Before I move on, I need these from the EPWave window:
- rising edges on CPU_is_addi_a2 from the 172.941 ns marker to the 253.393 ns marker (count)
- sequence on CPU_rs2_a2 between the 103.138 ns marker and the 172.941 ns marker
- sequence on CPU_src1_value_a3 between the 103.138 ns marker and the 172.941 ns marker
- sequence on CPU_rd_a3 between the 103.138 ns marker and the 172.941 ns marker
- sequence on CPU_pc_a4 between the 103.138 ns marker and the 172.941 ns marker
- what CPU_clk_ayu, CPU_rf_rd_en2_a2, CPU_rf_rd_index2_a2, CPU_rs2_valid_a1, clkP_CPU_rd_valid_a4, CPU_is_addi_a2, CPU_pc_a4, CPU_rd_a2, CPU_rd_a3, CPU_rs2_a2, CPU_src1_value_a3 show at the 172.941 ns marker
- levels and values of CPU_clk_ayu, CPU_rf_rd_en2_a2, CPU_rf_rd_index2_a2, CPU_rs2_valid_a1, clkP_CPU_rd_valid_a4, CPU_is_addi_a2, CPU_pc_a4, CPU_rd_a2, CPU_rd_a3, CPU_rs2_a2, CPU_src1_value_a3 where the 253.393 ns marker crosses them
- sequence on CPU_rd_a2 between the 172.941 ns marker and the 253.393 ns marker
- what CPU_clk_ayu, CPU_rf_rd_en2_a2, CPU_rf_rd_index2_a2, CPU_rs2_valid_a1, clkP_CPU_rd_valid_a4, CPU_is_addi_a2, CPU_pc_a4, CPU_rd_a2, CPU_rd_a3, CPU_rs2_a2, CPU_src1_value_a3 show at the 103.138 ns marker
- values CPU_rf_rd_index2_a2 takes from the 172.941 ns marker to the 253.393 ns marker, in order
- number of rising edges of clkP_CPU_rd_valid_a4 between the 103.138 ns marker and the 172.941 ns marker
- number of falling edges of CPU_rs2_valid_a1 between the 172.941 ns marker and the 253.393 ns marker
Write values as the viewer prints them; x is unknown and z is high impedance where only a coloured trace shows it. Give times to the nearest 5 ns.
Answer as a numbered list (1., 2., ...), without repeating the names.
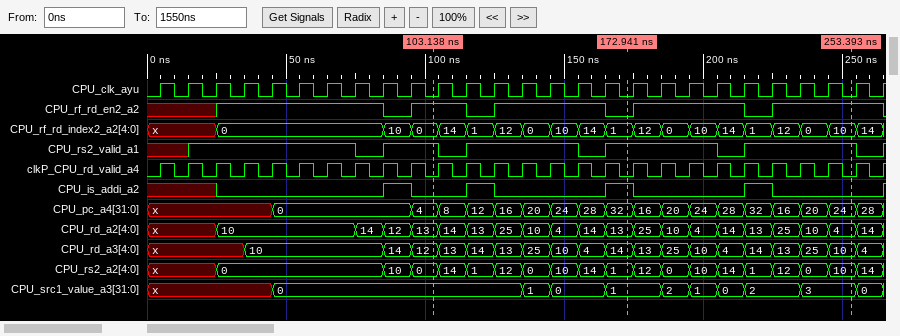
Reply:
1. 1
2. 0, 14, 1, 12, 0, 10, 14, 1
3. 0, 1, 0, 1
4. 12, 13, 14, 13, 25, 10, 4, 14
5. 4, 8, 12, 16, 20, 24, 28, 32
6. CPU_clk_ayu=0, CPU_rf_rd_en2_a2=0, CPU_rf_rd_index2_a2=1, CPU_rs2_valid_a1=1, clkP_CPU_rd_valid_a4=0, CPU_is_addi_a2=1, CPU_pc_a4=32, CPU_rd_a2=13, CPU_rd_a3=14, CPU_rs2_a2=1, CPU_src1_value_a3=1
7. CPU_clk_ayu=0, CPU_rf_rd_en2_a2=1, CPU_rf_rd_index2_a2=10, CPU_rs2_valid_a1=1, clkP_CPU_rd_valid_a4=0, CPU_is_addi_a2=0, CPU_pc_a4=24, CPU_rd_a2=4, CPU_rd_a3=10, CPU_rs2_a2=10, CPU_src1_value_a3=3
8. 13, 25, 10, 4, 14, 13, 25, 10, 4
9. CPU_clk_ayu=0, CPU_rf_rd_en2_a2=1, CPU_rf_rd_index2_a2=0, CPU_rs2_valid_a1=1, clkP_CPU_rd_valid_a4=0, CPU_is_addi_a2=0, CPU_pc_a4=4, CPU_rd_a2=13, CPU_rd_a3=12, CPU_rs2_a2=0, CPU_src1_value_a3=0
10. 1, 12, 0, 10, 14, 1, 12, 0, 10
11. 7
12. 1
